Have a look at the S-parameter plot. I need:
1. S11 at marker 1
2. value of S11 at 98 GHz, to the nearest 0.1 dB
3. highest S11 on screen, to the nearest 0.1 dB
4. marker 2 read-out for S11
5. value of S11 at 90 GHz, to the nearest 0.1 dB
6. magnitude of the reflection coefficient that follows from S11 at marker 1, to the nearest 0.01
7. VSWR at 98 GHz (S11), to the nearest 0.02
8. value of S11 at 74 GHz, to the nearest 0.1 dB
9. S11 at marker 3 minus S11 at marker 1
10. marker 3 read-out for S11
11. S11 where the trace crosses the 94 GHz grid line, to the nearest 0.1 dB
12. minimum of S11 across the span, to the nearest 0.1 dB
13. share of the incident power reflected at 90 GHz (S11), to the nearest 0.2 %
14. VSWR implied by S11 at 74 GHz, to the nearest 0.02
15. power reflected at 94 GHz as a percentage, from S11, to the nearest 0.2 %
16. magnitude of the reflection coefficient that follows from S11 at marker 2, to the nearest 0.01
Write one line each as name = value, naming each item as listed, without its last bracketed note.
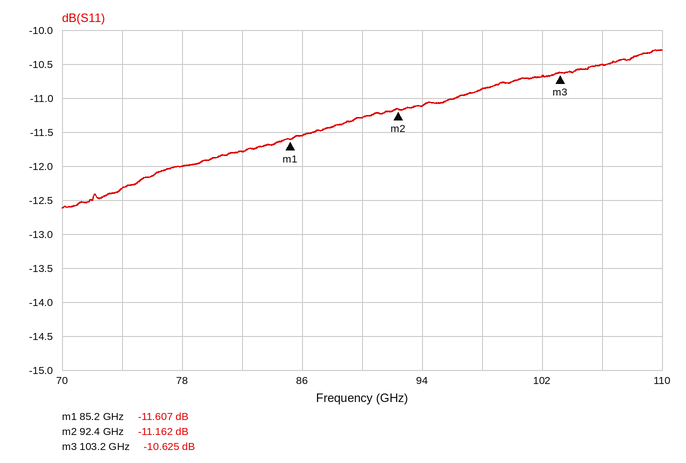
S11 at marker 1 = -11.607 dB
value of S11 at 98 GHz, to the nearest 0.1 dB = -10.9 dB
highest S11 on screen, to the nearest 0.1 dB = -10.3 dB
marker 2 read-out for S11 = -11.162 dB
value of S11 at 90 GHz, to the nearest 0.1 dB = -11.3 dB
magnitude of the reflection coefficient that follows from S11 at marker 1, to the nearest 0.01 = 0.26
VSWR at 98 GHz (S11), to the nearest 0.02 = 1.80
value of S11 at 74 GHz, to the nearest 0.1 dB = -12.3 dB
S11 at marker 3 minus S11 at marker 1 = 0.982 dB
marker 3 read-out for S11 = -10.625 dB
S11 where the trace crosses the 94 GHz grid line, to the nearest 0.1 dB = -11.1 dB
minimum of S11 across the span, to the nearest 0.1 dB = -12.6 dB
share of the incident power reflected at 90 GHz (S11), to the nearest 0.2 % = 7.4 %
VSWR implied by S11 at 74 GHz, to the nearest 0.02 = 1.64
power reflected at 94 GHz as a percentage, from S11, to the nearest 0.2 % = 7.8 %
magnitude of the reflection coefficient that follows from S11 at marker 2, to the nearest 0.01 = 0.28
